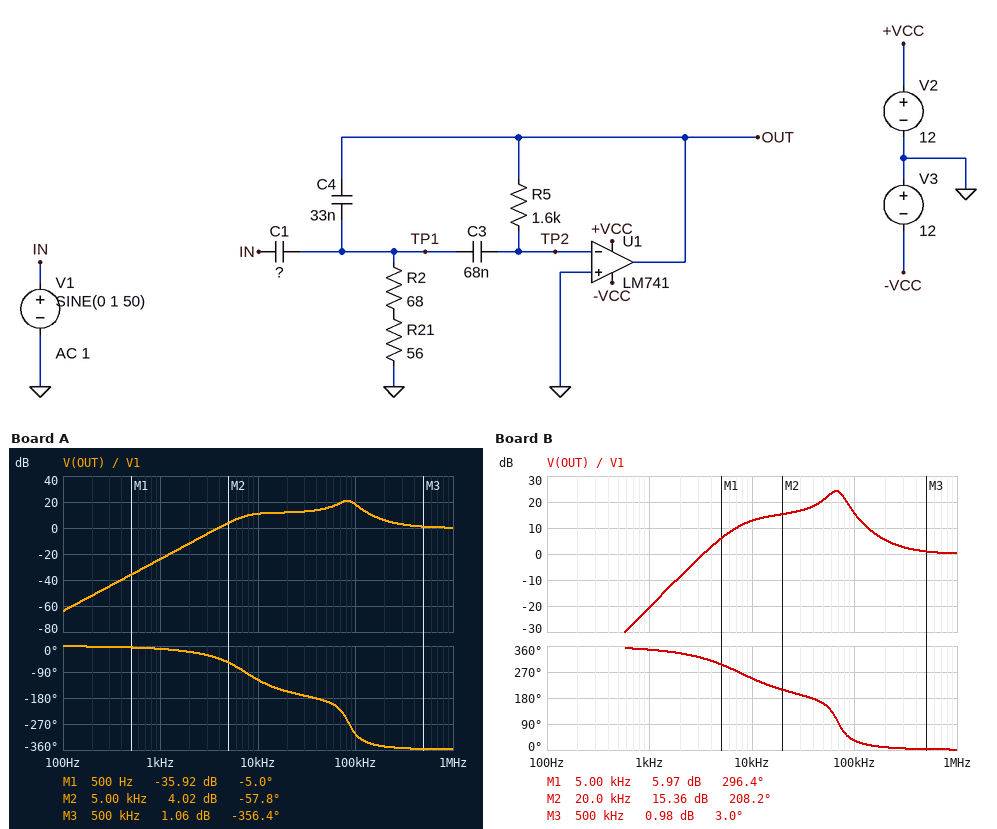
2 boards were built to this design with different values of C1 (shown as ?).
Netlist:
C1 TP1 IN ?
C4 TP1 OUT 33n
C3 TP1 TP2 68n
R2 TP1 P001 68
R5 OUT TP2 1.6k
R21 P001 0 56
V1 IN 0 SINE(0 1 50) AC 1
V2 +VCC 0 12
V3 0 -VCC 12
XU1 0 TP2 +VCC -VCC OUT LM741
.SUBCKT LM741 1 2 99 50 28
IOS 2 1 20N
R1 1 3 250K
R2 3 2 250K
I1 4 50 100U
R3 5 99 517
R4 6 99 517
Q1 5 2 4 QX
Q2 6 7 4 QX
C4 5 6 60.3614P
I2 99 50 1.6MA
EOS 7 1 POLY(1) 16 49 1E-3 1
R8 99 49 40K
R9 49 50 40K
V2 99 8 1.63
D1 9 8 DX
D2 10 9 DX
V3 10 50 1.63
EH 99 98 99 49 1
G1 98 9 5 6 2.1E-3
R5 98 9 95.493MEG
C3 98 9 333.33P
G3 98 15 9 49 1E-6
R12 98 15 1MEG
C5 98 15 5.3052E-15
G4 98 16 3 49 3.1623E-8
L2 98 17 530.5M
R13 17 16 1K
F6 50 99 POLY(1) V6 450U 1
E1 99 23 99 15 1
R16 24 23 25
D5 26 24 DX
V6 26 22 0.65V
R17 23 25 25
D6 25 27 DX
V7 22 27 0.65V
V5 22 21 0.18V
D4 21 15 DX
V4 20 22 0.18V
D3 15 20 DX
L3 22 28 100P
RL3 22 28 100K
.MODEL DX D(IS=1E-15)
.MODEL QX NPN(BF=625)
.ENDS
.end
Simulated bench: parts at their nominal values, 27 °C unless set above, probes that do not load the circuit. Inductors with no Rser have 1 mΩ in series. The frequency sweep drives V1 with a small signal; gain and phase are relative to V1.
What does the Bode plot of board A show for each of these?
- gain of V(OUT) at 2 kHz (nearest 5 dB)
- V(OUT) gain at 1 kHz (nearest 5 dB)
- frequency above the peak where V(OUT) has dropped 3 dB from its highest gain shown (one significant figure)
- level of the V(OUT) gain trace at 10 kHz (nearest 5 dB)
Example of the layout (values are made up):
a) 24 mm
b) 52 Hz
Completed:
a) -10 dB
b) -25 dB
c) 100 kHz
d) 10 dB
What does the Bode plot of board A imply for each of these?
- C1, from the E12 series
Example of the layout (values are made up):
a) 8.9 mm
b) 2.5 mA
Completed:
a) 120 nF
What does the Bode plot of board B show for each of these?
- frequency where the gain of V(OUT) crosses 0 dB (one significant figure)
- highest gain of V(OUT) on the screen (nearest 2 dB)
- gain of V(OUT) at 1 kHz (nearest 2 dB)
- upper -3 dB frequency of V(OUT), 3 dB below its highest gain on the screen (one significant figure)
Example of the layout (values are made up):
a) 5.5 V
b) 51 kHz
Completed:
a) 3 kHz
b) 24 dB
c) -20 dB
d) 80 kHz
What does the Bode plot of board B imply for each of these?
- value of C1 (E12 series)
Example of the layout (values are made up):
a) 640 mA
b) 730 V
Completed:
a) 180 nF
